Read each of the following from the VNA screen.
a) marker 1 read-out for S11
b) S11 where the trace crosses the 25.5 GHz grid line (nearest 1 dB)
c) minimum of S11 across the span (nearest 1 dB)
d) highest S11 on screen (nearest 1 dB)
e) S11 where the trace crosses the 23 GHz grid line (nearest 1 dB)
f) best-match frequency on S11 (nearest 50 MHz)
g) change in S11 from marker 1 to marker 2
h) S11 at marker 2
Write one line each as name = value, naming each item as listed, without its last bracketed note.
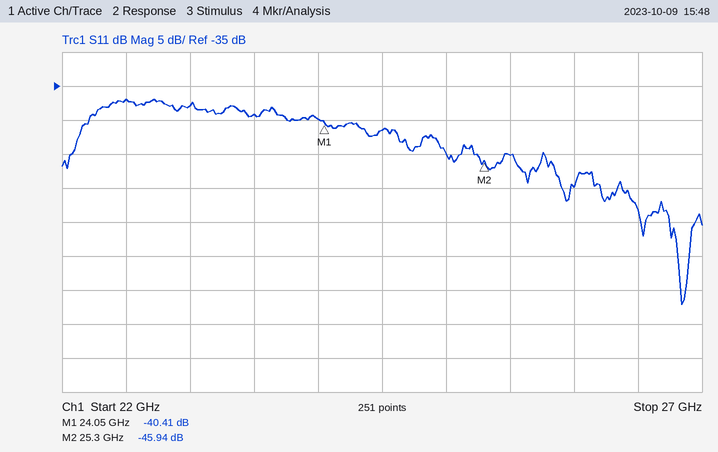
marker 1 read-out for S11 = -40.41 dB
S11 where the trace crosses the 25.5 GHz grid line = -45 dB
minimum of S11 across the span = -67 dB
highest S11 on screen = -37 dB
S11 where the trace crosses the 23 GHz grid line = -38 dB
best-match frequency on S11 = 26.85 GHz
change in S11 from marker 1 to marker 2 = -5.53 dB
S11 at marker 2 = -45.94 dB
